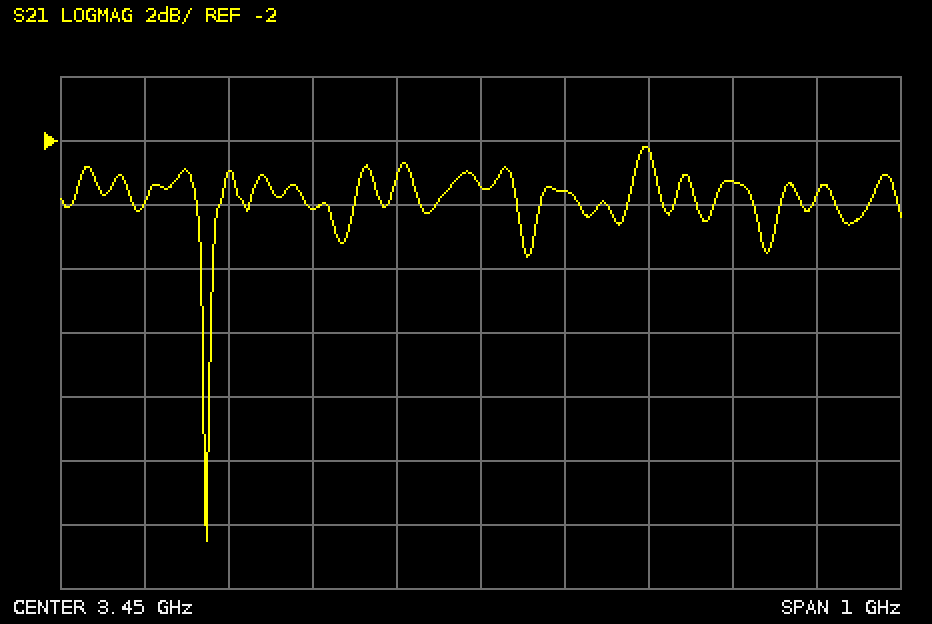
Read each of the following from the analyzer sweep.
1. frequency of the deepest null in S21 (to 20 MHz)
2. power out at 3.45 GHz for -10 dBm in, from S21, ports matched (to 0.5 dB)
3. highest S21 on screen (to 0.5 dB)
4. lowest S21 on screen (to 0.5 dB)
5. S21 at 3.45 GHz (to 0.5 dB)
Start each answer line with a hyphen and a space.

- 3.12 GHz
- -13.5 dBm
- -2.0 dB
- -14.5 dB
- -3.5 dB
